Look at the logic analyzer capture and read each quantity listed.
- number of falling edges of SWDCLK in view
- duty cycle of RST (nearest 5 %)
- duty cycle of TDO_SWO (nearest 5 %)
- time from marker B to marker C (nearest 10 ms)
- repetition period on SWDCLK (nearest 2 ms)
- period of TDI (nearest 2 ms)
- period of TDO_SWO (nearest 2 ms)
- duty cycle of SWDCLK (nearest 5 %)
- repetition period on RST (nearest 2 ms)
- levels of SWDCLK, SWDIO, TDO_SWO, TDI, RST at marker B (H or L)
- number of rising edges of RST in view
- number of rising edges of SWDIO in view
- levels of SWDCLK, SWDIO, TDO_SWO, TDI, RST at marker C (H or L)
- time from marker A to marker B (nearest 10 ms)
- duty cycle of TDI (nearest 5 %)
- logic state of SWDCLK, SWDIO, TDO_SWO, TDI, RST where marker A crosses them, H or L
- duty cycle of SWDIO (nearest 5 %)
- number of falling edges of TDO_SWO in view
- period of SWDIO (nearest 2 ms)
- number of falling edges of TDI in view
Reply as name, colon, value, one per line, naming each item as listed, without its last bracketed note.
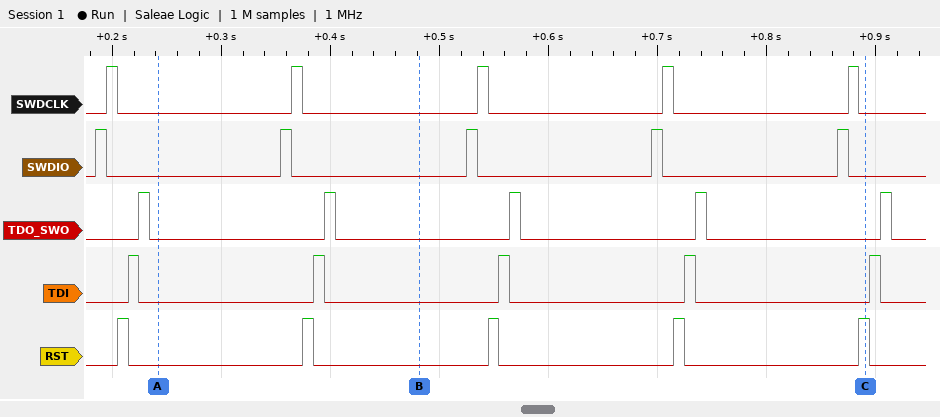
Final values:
number of falling edges of SWDCLK in view: 5
duty cycle of RST: 5 %
duty cycle of TDO_SWO: 5 %
time from marker B to marker C: 410 ms
repetition period on SWDCLK: 170 ms
period of TDI: 170 ms
period of TDO_SWO: 170 ms
duty cycle of SWDCLK: 5 %
repetition period on RST: 170 ms
levels of SWDCLK, SWDIO, TDO_SWO, TDI, RST at marker B: SWDCLK=L, SWDIO=L, TDO_SWO=L, TDI=L, RST=L
number of rising edges of RST in view: 5
number of rising edges of SWDIO in view: 5
levels of SWDCLK, SWDIO, TDO_SWO, TDI, RST at marker C: SWDCLK=L, SWDIO=L, TDO_SWO=L, TDI=L, RST=H
time from marker A to marker B: 240 ms
duty cycle of TDI: 5 %
logic state of SWDCLK, SWDIO, TDO_SWO, TDI, RST where marker A crosses them, H or L: SWDCLK=L, SWDIO=L, TDO_SWO=L, TDI=L, RST=L
duty cycle of SWDIO: 5 %
number of falling edges of TDO_SWO in view: 5
period of SWDIO: 170 ms
number of falling edges of TDI in view: 5
